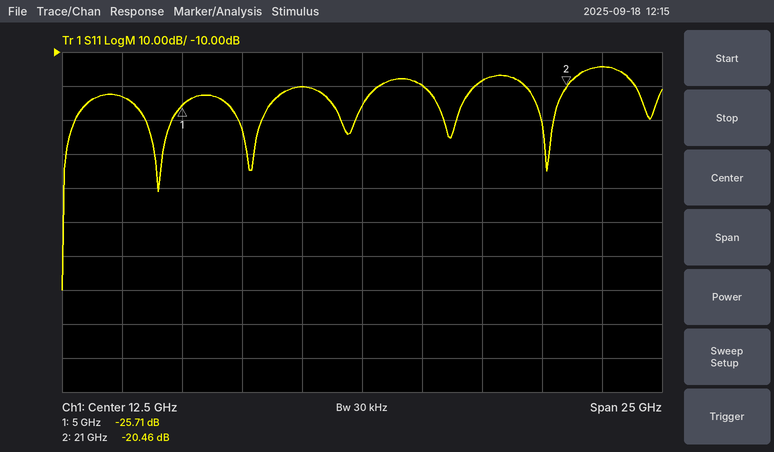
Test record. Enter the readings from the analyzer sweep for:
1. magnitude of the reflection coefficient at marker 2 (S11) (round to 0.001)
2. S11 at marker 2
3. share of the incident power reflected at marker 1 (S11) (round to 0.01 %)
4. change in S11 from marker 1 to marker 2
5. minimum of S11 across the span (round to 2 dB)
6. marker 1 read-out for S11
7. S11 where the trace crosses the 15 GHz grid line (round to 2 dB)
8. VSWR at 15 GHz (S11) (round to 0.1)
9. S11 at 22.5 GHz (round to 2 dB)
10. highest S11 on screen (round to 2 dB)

0.095
-20.46 dB
0.27 %
5.25 dB
-80 dB
-25.71 dB
-20 dB
1.2
-14 dB
-14 dB
